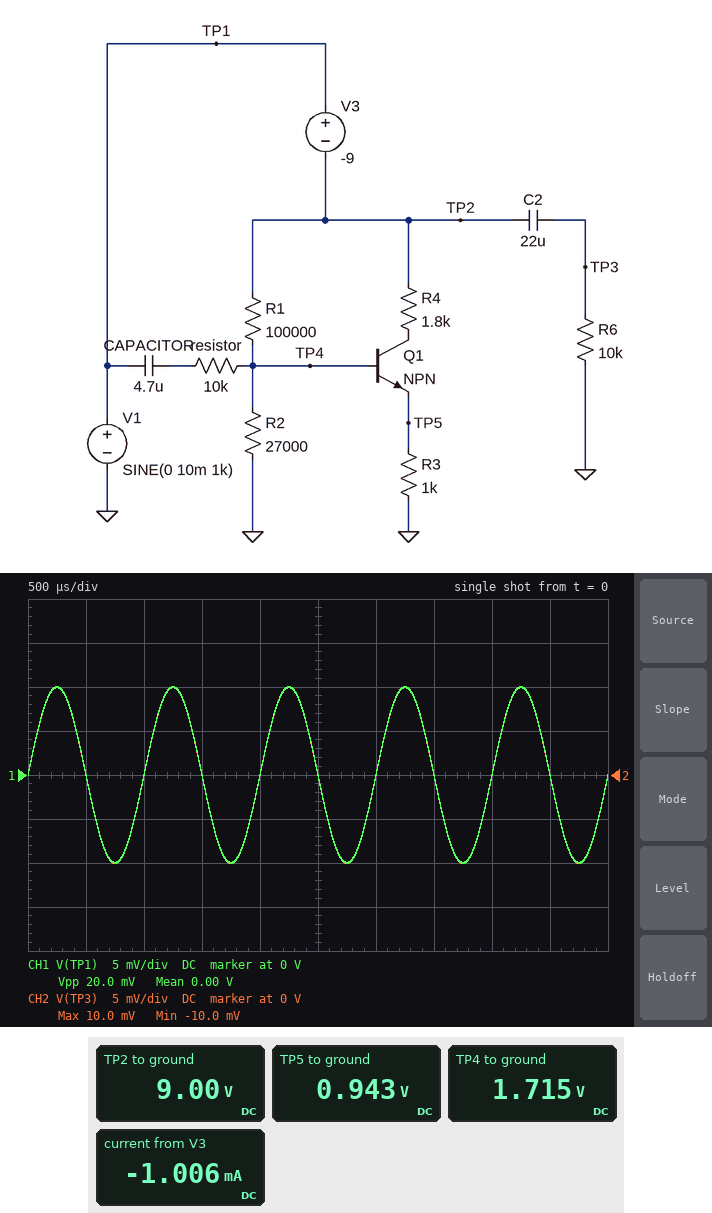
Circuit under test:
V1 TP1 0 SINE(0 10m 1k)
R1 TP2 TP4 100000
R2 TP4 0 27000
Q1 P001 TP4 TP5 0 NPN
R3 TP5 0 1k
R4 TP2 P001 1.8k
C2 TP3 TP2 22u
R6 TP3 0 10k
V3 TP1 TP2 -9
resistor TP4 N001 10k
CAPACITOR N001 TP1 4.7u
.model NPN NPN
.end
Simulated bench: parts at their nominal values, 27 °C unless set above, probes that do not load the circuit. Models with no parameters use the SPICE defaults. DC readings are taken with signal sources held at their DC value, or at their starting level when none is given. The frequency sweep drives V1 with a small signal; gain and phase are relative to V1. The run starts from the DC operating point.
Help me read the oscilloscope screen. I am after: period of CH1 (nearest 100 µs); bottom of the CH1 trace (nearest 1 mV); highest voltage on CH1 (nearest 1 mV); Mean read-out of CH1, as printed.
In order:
1.0 ms
-10 mV
10 mV
0.00 V
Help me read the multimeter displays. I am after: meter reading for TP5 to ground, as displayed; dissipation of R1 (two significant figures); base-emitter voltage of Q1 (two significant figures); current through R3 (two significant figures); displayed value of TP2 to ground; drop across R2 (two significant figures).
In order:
0.943 V
530 µW
770 mV
940 µA
9.00 V
1.7 V
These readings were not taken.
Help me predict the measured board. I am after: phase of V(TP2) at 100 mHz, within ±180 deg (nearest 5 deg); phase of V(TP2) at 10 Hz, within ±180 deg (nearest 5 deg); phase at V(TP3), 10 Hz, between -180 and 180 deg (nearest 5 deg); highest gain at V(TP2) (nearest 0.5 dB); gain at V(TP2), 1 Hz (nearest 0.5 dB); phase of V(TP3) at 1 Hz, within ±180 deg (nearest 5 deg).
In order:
0 deg
0 deg
5 deg
0 dB
0 dB
35 deg
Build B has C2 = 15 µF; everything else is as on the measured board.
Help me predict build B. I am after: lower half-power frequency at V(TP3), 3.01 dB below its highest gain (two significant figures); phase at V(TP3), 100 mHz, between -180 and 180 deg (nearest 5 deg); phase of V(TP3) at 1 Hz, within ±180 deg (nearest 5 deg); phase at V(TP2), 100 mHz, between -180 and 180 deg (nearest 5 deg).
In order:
1.1 Hz
85 deg
45 deg
0 deg
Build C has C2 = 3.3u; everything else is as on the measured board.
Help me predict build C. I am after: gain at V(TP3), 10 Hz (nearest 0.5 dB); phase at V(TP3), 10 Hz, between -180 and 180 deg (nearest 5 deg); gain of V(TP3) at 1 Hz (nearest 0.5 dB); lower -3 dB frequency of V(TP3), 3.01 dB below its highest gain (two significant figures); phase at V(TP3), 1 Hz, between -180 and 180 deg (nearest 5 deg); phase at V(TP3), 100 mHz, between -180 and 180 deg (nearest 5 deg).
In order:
-1.0 dB
25 deg
-14.0 dB
4.8 Hz
80 deg
90 deg
